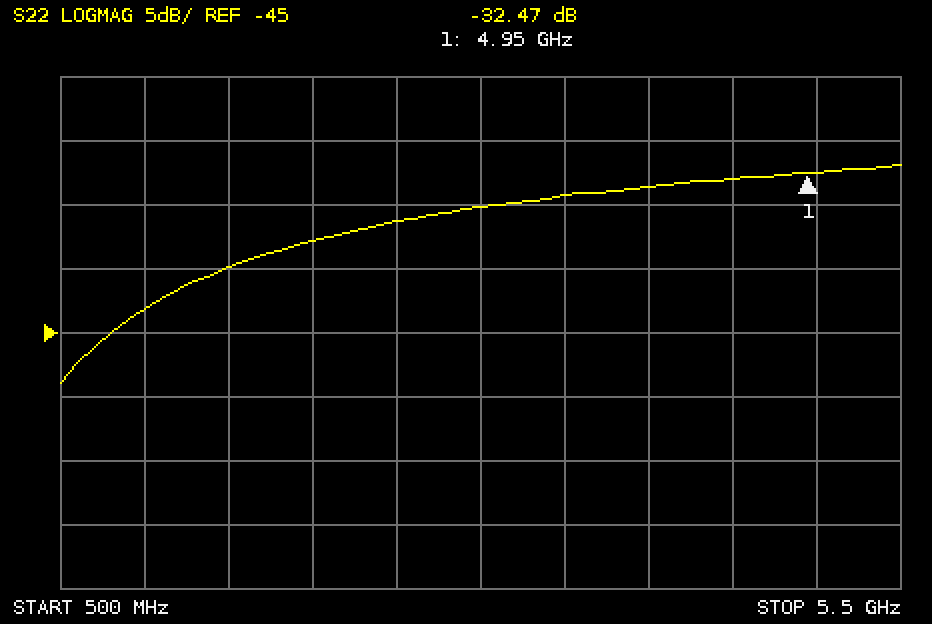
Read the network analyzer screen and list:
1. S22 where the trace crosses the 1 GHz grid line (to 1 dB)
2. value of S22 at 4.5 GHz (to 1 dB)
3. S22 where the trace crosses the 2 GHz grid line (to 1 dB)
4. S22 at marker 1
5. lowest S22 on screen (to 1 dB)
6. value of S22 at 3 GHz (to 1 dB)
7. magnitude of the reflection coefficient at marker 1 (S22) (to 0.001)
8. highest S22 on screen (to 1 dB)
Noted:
-43 dB
-33 dB
-38 dB
-32.47 dB
-49 dB
-35 dB
0.024
-32 dB
